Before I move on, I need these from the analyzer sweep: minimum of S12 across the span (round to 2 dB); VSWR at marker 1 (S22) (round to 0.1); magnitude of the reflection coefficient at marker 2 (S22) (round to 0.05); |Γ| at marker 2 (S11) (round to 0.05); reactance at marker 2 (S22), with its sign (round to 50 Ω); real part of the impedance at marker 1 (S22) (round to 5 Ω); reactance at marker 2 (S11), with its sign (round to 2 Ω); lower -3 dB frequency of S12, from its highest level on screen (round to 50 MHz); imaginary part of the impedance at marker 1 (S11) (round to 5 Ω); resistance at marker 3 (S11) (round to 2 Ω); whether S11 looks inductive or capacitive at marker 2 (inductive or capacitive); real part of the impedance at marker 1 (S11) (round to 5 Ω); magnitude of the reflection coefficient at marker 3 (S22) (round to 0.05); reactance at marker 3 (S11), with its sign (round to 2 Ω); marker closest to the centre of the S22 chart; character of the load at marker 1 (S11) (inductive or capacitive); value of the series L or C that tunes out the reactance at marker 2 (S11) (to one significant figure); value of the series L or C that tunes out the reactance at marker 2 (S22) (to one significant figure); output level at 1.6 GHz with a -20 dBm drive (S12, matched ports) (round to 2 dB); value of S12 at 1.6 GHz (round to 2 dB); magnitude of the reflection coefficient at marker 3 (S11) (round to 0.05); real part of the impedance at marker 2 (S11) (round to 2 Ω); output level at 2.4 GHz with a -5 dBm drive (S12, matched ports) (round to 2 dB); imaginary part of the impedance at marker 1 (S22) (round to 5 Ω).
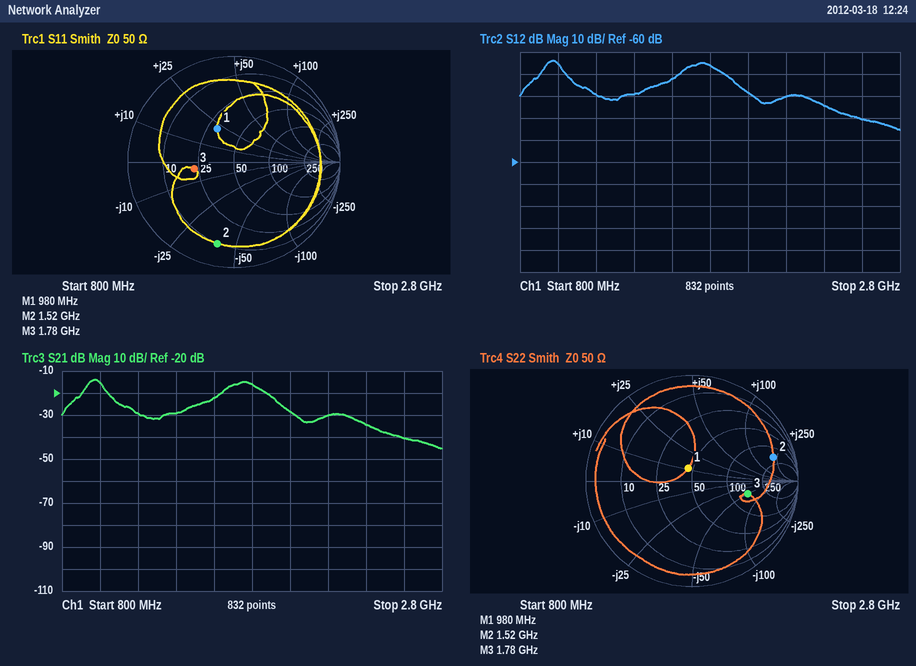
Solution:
-46 dB
1.3
0.80
0.80
+200 Ω
45 Ω
-40 Ω
950 MHz
+20 Ω
22 Ω
capacitive
30 Ω
0.55
-4 Ω
marker 1
inductive
4 nH
500 fF
-42 dBm
-22 dB
0.40
10 Ω
-40 dBm
+10 Ω
